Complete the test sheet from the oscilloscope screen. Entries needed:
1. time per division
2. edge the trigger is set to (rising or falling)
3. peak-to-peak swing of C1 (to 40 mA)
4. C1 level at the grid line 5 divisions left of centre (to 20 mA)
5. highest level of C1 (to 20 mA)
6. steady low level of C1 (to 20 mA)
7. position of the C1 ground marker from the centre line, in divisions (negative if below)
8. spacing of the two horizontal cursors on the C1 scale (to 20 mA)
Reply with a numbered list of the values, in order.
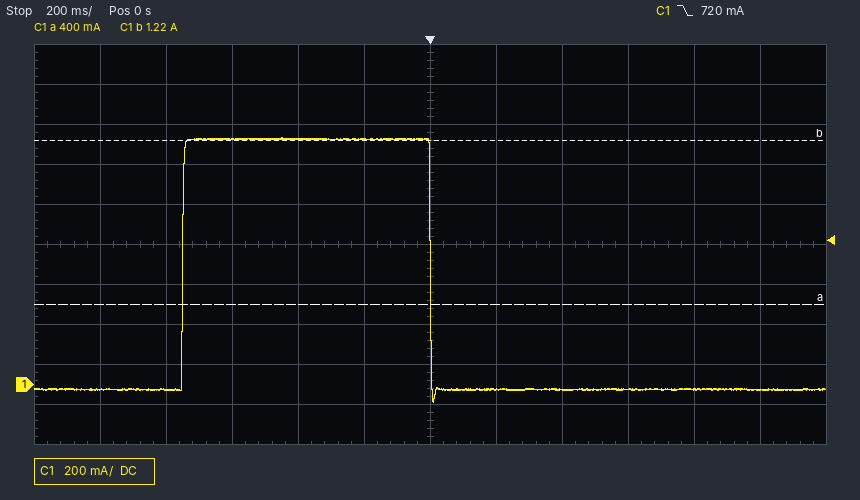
1. 200 ms
2. falling
3. 1.32 A
4. -20 mA
5. 1.24 A
6. -20 mA
7. -3.5 div
8. 820 mA
